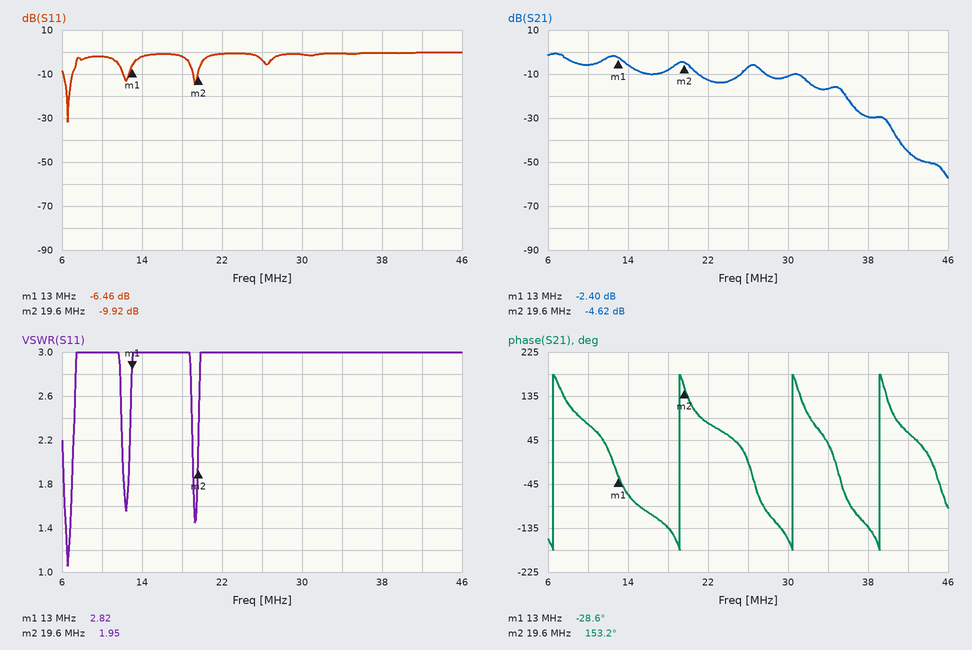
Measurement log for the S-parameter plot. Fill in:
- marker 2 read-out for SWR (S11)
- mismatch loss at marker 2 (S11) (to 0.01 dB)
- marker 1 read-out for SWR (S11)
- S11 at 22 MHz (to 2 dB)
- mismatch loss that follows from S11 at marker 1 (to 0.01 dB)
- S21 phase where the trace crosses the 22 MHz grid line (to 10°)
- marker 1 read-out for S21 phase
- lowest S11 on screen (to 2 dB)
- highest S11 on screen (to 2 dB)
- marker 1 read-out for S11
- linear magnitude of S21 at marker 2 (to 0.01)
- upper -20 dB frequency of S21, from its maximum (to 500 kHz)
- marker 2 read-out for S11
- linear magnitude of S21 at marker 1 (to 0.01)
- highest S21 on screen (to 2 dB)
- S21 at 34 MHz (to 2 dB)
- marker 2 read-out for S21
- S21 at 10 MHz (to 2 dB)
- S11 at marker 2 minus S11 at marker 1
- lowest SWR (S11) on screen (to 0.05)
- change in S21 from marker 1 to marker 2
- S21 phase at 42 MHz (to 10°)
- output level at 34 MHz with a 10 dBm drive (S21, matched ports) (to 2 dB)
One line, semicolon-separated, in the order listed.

1.95; 0.47 dB; 2.82; 0 dB; 1.11 dB; 80°; -28.6°; -32 dB; 0 dB; -6.46 dB; 0.59; 36.0 MHz; -9.92 dB; 0.76; 0 dB; -16 dB; -4.62 dB; -6 dB; -3.46 dB; 1.05; -2.22 dB; 60°; -6 dBm
